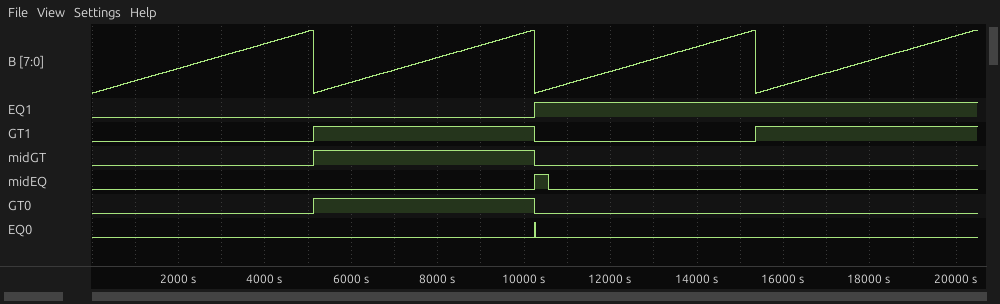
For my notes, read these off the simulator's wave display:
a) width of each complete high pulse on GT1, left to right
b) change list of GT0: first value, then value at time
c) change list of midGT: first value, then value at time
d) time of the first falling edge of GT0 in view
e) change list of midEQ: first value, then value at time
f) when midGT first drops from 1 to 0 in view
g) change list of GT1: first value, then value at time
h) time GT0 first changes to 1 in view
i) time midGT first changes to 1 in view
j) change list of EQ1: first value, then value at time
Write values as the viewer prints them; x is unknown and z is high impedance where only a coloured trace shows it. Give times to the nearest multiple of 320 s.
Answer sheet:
5120 s
0, 1 at 5120 s, 0 at 10240 s
0, 1 at 5120 s, 0 at 10240 s
10240 s
0, 1 at 10240 s, 0 at 10560 s
10240 s
0, 1 at 5120 s, 0 at 10240 s, 1 at 15360 s
5120 s
5120 s
0, 1 at 10240 s
